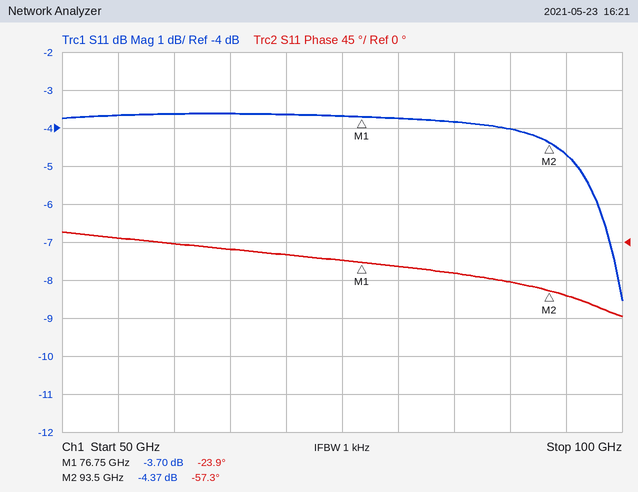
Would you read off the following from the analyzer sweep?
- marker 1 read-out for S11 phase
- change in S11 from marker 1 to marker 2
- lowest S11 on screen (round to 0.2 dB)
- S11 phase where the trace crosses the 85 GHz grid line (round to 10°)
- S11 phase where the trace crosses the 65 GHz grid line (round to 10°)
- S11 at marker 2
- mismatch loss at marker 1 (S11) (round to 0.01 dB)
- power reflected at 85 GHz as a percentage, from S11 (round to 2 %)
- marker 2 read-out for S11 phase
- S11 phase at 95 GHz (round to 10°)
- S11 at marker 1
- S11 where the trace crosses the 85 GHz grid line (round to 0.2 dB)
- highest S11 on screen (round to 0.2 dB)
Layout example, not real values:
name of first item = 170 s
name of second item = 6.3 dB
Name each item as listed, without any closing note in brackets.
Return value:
marker 1 read-out for S11 phase = -23.9°
change in S11 from marker 1 to marker 2 = -0.67 dB
lowest S11 on screen = -8.6 dB
S11 phase where the trace crosses the 85 GHz grid line = -40°
S11 phase where the trace crosses the 65 GHz grid line = -10°
S11 at marker 2 = -4.37 dB
mismatch loss at marker 1 (S11) = 2.42 dB
power reflected at 85 GHz as a percentage, from S11 = 42 %
marker 2 read-out for S11 phase = -57.3°
S11 phase at 95 GHz = -60°
S11 at marker 1 = -3.70 dB
S11 where the trace crosses the 85 GHz grid line = -3.8 dB
highest S11 on screen = -3.6 dB
